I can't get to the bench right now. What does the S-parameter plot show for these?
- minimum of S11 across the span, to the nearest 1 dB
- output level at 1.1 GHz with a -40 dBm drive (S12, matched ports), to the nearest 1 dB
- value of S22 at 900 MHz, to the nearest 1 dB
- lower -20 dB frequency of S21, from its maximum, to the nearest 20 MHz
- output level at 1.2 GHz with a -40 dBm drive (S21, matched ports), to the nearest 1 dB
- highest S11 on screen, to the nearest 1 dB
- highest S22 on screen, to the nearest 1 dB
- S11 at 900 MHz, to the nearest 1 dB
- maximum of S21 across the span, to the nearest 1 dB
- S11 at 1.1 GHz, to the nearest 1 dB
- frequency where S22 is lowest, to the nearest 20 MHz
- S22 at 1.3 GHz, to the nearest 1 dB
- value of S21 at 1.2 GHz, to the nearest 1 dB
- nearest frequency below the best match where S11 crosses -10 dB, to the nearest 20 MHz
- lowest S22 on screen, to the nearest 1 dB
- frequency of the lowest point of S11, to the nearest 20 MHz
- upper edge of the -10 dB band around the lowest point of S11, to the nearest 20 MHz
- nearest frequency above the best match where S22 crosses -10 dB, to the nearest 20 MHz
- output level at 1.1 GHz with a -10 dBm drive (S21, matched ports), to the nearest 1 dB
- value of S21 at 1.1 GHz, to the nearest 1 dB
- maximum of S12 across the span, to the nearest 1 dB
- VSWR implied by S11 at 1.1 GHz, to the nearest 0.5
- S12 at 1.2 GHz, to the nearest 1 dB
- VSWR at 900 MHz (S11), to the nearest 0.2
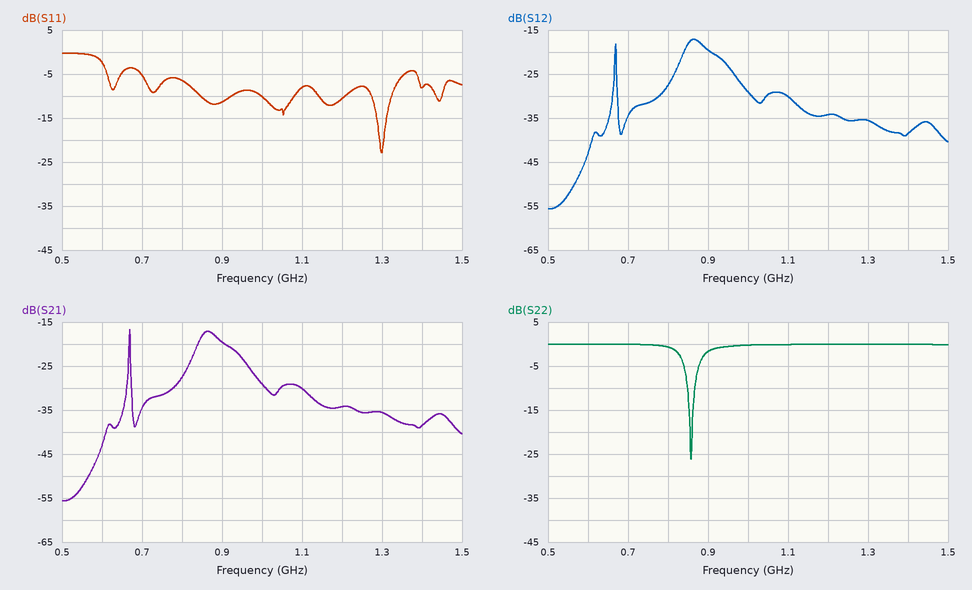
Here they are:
-23 dB
-70 dBm
-2 dB
640 MHz
-74 dBm
0 dB
0 dB
-11 dB
-17 dB
-8 dB
860 MHz
0 dB
-34 dB
1.28 GHz
-26 dB
1.30 GHz
1.32 GHz
860 MHz
-40 dBm
-30 dB
-17 dB
2.5
-34 dB
1.8
